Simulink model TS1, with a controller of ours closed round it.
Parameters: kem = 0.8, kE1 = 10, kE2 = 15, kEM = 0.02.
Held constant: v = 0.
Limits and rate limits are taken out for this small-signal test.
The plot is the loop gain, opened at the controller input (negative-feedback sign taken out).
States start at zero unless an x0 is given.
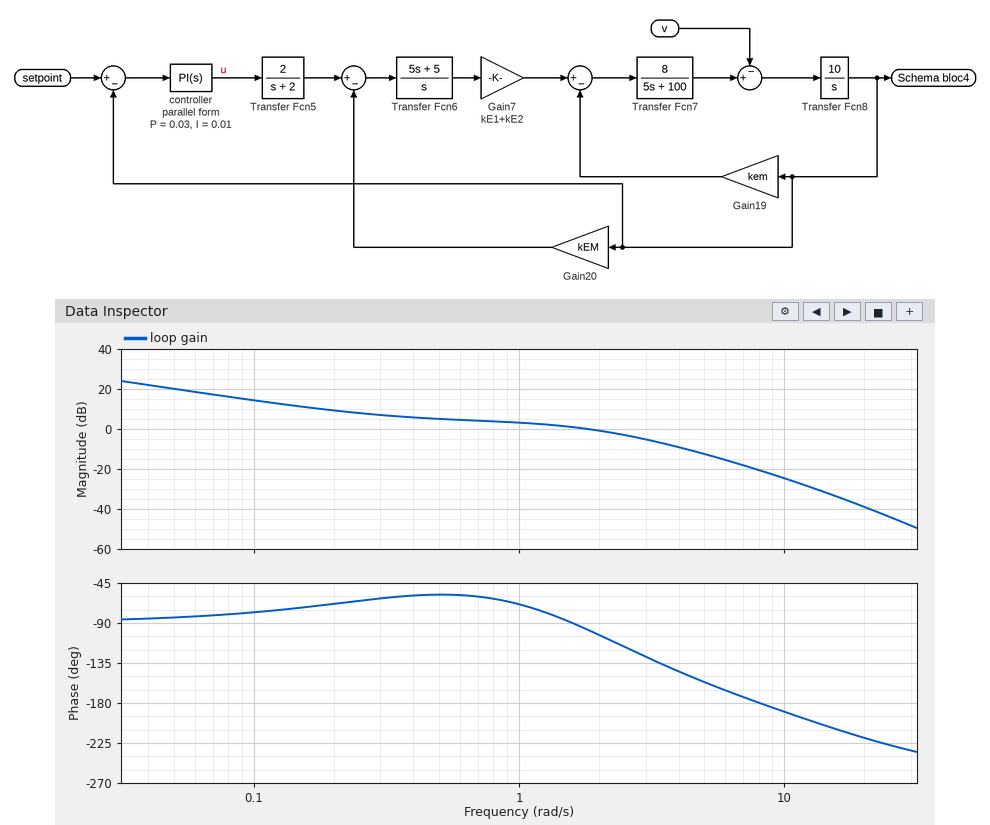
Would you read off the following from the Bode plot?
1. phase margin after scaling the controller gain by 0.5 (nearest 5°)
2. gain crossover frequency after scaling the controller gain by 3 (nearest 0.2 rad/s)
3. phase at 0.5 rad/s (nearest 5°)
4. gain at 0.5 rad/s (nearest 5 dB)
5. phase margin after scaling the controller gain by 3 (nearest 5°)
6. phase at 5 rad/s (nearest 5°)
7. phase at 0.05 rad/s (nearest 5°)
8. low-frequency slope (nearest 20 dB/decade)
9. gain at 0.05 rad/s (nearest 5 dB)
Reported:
120°
4.2 rad/s
-60°
5 dB
35°
-155°
-85°
-20 dB/decade
20 dB
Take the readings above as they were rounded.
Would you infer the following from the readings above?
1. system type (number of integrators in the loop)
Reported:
1
